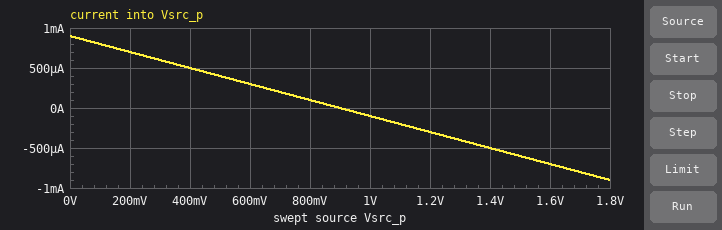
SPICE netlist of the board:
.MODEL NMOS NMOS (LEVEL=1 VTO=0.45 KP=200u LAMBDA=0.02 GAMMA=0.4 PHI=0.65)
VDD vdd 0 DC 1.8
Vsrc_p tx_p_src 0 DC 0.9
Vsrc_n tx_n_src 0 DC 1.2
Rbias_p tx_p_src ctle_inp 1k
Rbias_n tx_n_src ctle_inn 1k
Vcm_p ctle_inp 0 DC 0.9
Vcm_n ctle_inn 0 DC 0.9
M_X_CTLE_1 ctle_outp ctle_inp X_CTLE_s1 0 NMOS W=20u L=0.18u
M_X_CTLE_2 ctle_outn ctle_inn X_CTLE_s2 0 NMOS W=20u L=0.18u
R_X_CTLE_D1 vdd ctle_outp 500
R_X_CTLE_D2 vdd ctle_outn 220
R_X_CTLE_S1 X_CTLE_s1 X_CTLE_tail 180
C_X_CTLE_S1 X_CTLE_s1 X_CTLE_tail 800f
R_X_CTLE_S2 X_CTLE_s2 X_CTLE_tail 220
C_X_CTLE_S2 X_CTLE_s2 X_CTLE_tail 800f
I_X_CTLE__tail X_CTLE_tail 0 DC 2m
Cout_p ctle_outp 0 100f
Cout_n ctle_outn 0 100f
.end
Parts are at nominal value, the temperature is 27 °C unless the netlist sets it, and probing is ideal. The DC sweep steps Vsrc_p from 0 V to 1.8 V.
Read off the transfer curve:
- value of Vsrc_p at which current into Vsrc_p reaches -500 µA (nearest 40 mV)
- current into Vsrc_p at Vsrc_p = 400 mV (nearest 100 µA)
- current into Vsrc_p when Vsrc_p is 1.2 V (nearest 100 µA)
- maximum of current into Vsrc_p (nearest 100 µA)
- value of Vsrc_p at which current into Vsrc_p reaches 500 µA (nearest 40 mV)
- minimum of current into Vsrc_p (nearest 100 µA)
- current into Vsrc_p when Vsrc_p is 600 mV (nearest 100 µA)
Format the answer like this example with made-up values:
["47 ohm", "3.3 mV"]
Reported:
["1.40 V", "500 µA", "-300 µA", "900 µA", "400 mV", "-900 µA", "300 µA"]
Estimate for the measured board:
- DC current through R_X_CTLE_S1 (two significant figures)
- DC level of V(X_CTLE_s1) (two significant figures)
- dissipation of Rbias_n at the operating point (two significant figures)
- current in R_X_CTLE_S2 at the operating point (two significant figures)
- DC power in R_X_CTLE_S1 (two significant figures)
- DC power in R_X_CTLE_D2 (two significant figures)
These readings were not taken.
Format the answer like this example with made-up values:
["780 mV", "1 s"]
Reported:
["1.1 mA", "120 mV", "90 µW", "940 µA", "200 µW", "190 µW"]
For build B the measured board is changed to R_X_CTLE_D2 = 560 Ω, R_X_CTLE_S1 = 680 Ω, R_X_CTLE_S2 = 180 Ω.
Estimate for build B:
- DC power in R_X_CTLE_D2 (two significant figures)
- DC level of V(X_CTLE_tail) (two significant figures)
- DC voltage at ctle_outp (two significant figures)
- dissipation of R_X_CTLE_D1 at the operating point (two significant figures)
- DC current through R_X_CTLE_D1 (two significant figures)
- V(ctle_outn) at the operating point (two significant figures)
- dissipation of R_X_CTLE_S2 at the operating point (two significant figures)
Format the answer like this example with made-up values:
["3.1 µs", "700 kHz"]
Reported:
["1.2 mW", "-190 mV", "1.5 V", "150 µW", "550 µA", "990 mV", "380 µW"]
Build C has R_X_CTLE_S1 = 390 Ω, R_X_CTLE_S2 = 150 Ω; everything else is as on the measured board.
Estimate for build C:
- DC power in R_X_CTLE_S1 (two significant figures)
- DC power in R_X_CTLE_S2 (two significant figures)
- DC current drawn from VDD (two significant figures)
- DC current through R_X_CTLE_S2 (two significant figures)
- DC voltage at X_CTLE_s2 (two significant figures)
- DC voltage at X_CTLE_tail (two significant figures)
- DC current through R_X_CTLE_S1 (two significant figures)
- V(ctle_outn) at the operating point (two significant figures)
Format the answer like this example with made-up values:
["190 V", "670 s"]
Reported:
["190 µW", "260 µW", "2.0 mA", "1.3 mA", "90 mV", "-110 mV", "690 µA", "1.5 V"]
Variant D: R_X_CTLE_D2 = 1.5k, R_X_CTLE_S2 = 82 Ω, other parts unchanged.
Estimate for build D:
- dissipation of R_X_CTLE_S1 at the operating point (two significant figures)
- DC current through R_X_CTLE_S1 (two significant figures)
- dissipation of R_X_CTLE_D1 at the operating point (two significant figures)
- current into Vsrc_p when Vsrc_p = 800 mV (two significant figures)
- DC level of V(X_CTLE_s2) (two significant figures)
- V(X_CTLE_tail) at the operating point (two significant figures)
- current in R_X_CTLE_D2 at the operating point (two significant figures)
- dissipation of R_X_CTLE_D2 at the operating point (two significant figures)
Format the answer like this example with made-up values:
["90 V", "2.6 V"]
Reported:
["160 µW", "940 µA", "440 µW", "100 µA", "51 mV", "-37 mV", "1.1 mA", "1.7 mW"]
